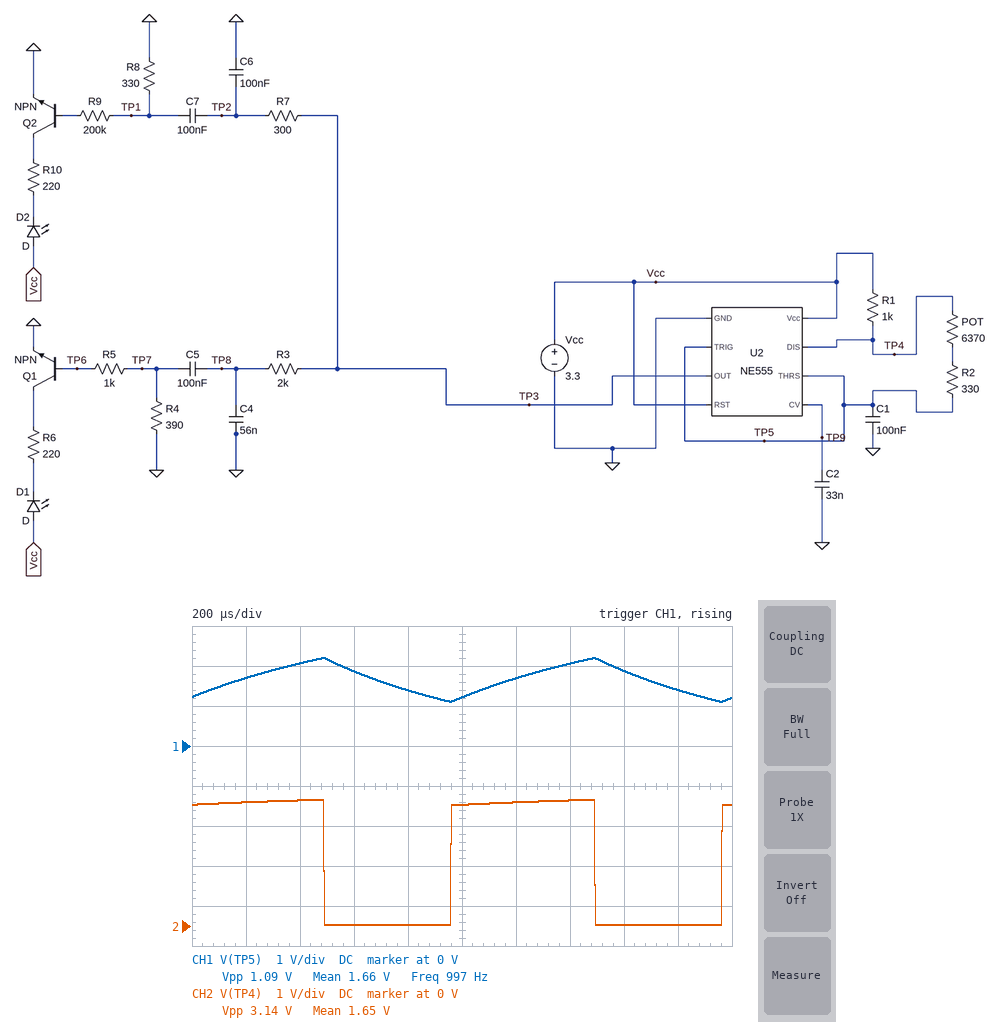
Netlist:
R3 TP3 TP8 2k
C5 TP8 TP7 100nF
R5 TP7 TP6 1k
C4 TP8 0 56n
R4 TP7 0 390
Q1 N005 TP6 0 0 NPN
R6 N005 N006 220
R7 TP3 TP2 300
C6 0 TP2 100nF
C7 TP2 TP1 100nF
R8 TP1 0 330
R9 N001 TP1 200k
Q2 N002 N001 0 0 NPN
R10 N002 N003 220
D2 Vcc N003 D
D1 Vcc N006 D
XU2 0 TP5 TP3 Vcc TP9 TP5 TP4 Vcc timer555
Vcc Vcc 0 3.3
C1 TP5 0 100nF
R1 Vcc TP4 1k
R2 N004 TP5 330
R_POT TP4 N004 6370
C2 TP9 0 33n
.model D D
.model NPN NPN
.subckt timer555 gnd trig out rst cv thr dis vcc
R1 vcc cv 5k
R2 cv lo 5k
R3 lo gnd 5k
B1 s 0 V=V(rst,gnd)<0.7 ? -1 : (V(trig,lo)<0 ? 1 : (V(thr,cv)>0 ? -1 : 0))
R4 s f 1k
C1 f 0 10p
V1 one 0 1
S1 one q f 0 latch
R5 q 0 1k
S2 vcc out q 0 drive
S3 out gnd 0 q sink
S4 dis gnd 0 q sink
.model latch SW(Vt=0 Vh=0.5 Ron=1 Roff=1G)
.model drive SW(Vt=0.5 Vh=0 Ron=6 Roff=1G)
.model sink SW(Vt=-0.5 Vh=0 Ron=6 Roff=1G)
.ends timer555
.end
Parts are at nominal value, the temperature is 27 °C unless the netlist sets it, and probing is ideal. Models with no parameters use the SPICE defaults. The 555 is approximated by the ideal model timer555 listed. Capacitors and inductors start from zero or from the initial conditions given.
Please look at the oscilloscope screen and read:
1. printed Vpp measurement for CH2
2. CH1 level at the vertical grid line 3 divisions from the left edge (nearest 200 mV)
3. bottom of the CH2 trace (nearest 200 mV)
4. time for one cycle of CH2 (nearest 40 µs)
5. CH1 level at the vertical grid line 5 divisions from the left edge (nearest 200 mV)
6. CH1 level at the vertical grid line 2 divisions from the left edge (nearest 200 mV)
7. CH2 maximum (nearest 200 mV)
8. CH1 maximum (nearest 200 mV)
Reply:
3.14 V
1.8 V
0 V
1.00 ms
1.2 V
2.0 V
3.2 V
2.2 V
